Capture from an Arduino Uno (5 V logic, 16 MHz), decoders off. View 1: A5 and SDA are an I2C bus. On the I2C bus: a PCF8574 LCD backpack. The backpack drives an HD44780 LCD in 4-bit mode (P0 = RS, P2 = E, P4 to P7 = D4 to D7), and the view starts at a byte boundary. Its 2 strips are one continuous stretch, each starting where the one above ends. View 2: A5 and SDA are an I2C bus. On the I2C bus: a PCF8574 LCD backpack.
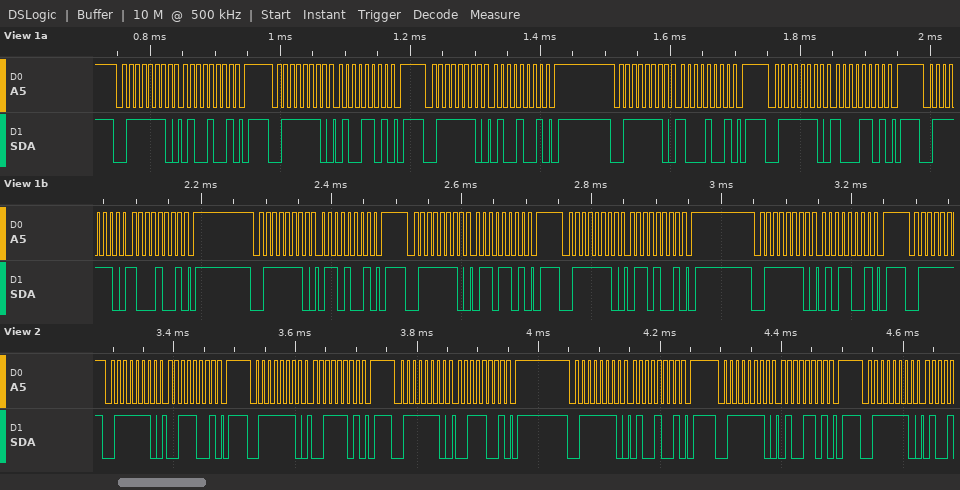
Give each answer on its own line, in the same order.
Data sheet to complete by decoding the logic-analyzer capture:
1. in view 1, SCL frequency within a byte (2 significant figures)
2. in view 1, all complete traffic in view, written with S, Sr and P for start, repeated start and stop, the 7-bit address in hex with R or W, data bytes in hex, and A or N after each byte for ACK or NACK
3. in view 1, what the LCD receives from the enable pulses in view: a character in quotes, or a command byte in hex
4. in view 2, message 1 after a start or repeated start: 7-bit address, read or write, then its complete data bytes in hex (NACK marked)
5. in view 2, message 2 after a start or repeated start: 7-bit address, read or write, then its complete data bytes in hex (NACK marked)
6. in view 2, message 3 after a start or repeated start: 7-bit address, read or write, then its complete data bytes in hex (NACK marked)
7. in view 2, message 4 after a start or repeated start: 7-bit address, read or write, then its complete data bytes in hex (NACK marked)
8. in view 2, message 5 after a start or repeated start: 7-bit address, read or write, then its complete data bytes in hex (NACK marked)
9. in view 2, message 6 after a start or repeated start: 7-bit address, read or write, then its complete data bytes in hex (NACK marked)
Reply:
100 kHz
S 3FW A 49 A P S 3FW A 4D A P S 3FW A 49 A P S 3FW A 89 A P S 3FW A 8D A P S 3FW A 89 A P S 3FW A 69 A P S 3FW A 6D A P S 3FW A 69 A P S 3FW A 59 A P
'H'
0x3F write: 39
0x3F write: 3D
0x3F write: 39
0x3F write: 49
0x3F write: 4D
0x3F write
